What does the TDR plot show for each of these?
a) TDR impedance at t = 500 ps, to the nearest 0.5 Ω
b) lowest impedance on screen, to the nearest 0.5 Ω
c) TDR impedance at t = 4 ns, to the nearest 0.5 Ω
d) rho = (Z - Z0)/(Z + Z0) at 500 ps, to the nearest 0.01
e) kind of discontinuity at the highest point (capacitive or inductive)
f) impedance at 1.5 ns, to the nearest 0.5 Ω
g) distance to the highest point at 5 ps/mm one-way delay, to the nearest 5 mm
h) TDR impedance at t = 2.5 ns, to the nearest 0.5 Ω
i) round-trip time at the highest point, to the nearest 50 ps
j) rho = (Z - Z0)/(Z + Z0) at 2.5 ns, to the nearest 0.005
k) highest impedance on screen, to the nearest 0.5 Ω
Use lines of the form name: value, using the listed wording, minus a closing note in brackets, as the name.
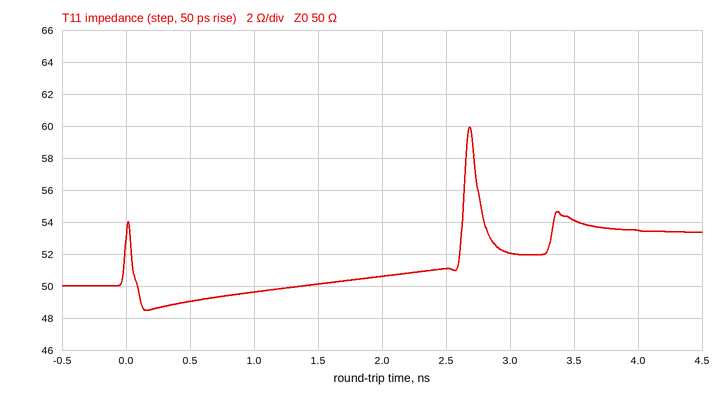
TDR impedance at t = 500 ps, to the nearest 0.5 Ω: 49.0 Ω
lowest impedance on screen, to the nearest 0.5 Ω: 48.5 Ω
TDR impedance at t = 4 ns, to the nearest 0.5 Ω: 53.5 Ω
rho = (Z - Z0)/(Z + Z0) at 500 ps, to the nearest 0.01: -0.01
kind of discontinuity at the highest point: inductive
impedance at 1.5 ns, to the nearest 0.5 Ω: 50.0 Ω
distance to the highest point at 5 ps/mm one-way delay, to the nearest 5 mm: 270 mm
TDR impedance at t = 2.5 ns, to the nearest 0.5 Ω: 51.0 Ω
round-trip time at the highest point, to the nearest 50 ps: 2.70 ns
rho = (Z - Z0)/(Z + Z0) at 2.5 ns, to the nearest 0.005: +0.010
highest impedance on screen, to the nearest 0.5 Ω: 60.0 Ω
